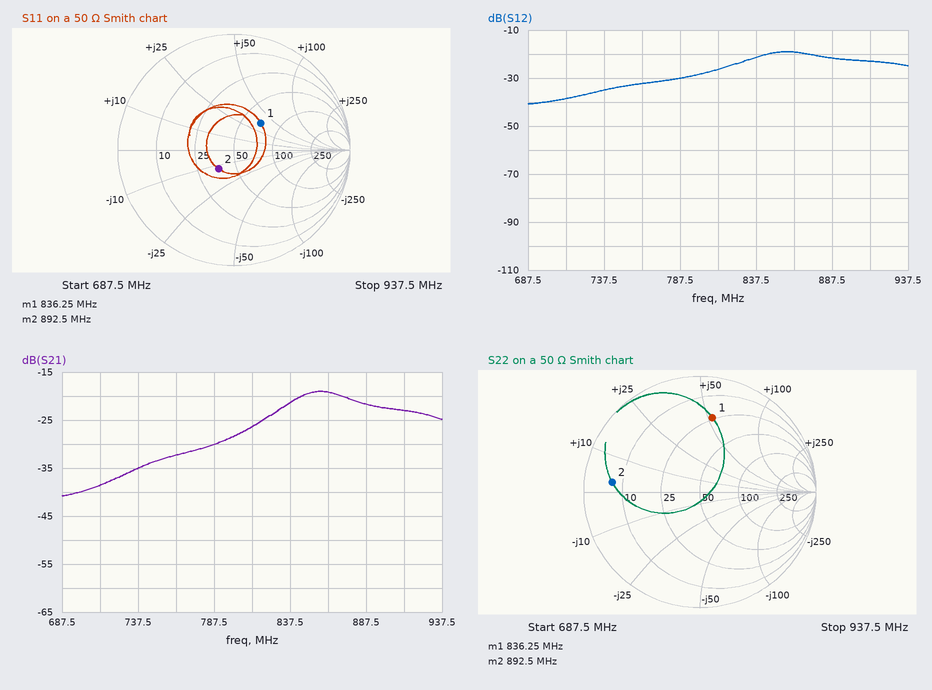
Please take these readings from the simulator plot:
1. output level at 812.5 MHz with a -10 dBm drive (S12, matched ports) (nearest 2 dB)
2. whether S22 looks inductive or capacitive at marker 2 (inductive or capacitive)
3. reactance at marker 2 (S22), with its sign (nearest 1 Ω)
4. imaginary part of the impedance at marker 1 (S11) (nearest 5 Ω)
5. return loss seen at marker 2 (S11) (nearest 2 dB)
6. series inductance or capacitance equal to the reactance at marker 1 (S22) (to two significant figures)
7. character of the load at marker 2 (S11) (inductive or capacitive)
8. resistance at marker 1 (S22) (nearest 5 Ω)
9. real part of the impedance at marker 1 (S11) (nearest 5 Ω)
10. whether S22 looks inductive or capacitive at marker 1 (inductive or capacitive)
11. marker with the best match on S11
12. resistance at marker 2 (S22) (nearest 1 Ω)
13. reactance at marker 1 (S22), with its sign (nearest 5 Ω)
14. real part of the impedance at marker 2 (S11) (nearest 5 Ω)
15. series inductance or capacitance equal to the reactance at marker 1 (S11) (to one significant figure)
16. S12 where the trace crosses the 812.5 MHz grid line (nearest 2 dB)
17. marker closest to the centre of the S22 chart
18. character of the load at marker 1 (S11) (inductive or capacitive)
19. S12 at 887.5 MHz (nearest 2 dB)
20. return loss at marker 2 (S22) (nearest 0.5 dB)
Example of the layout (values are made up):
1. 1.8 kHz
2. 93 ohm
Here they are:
1. -36 dBm
2. inductive
3. +3 Ω
4. +35 Ω
5. 14 dB
6. 10 nH
7. capacitive
8. 25 Ω
9. 70 Ω
10. inductive
11. marker 2
12. 7 Ω
13. +55 Ω
14. 35 Ω
15. 7 nH
16. -26 dB
17. marker 1
18. inductive
19. -22 dB
20. 2.5 dB
